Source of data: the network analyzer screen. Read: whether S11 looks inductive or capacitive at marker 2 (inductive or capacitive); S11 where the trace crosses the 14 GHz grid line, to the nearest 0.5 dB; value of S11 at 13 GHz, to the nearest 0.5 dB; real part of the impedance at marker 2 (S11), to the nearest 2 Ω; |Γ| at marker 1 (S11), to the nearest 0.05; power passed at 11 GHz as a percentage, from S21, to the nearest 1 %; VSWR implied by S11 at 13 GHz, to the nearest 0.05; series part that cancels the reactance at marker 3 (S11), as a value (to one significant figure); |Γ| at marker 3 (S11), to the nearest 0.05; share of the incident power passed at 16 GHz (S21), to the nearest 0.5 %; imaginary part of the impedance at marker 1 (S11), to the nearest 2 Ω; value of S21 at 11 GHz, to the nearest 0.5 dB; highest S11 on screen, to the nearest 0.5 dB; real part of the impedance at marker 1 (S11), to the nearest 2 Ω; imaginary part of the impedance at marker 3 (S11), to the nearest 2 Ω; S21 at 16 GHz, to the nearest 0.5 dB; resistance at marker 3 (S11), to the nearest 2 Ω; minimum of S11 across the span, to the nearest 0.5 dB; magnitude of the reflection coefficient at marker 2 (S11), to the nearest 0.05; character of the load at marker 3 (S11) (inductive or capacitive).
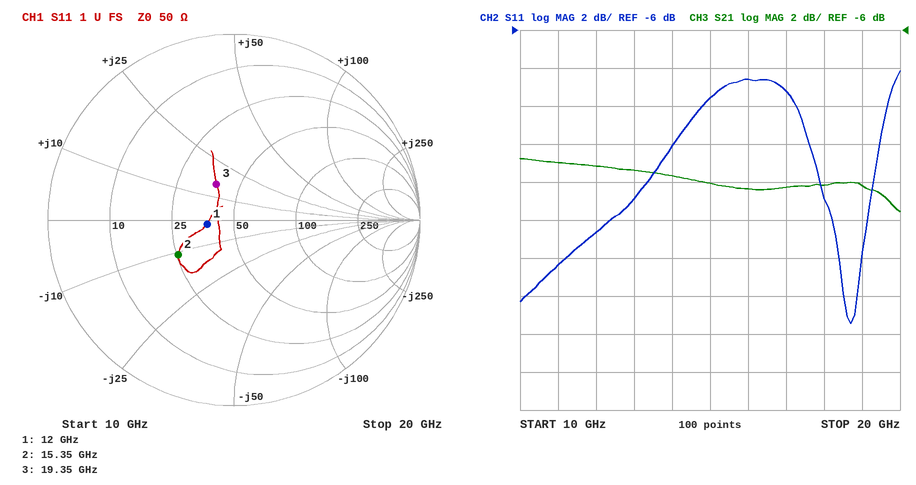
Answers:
capacitive
-12.0 dB
-15.0 dB
26 Ω
0.15
5 %
1.45
500 fF
0.20
3.5 %
-2 Ω
-13.0 dB
-8.0 dB
38 Ω
+16 Ω
-14.5 dB
38 Ω
-21.5 dB
0.35
inductive
